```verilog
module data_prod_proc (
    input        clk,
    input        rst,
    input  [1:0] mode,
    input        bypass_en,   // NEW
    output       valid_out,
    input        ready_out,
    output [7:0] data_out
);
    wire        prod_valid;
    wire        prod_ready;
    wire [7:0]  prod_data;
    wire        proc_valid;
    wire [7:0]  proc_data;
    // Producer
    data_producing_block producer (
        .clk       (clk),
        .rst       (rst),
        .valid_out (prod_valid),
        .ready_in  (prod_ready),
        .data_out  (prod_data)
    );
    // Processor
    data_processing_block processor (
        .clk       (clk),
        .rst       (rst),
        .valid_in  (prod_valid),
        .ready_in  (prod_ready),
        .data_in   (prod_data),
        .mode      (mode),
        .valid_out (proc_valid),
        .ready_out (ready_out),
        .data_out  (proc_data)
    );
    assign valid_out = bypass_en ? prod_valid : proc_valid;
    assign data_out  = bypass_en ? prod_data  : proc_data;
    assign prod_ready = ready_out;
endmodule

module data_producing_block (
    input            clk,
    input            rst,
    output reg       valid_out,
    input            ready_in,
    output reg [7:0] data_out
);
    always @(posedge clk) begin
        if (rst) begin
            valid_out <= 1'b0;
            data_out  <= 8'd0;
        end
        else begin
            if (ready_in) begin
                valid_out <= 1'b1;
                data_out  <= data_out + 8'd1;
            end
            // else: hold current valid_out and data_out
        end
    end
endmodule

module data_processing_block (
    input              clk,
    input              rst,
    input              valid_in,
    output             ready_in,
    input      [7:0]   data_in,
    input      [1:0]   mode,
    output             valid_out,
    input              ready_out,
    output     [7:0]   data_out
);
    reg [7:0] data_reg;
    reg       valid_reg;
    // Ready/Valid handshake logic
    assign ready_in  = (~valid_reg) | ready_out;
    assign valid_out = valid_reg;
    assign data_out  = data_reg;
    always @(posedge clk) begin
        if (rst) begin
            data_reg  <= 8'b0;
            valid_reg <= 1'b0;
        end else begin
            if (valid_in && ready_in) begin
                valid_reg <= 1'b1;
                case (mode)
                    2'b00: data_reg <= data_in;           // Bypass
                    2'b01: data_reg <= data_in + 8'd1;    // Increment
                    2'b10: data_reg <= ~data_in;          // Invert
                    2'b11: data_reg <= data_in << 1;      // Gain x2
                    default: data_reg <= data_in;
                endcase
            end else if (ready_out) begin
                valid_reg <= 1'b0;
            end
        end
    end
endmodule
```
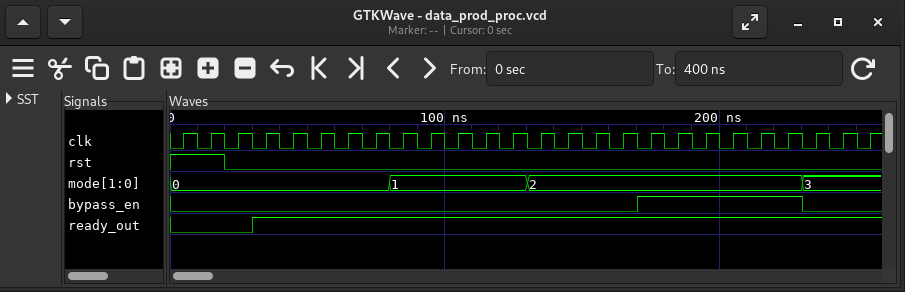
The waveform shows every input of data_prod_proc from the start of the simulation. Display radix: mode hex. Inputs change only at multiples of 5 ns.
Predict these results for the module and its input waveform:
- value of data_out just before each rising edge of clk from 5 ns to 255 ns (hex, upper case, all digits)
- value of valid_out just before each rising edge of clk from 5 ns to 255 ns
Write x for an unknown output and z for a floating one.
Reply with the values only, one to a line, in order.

x, 00, 00, 00, 00, 01, 02, 03, 04, 06, 07, 08, 09, 0A, F5, F4, F3, 0E, 0F, 10, 11, 12, 13, EC, 28, 2A
x 0 0 0 0 1 1 1 1 1 1 1 1 1 1 1 1 1 1 1 1 1 1 1 1 1
